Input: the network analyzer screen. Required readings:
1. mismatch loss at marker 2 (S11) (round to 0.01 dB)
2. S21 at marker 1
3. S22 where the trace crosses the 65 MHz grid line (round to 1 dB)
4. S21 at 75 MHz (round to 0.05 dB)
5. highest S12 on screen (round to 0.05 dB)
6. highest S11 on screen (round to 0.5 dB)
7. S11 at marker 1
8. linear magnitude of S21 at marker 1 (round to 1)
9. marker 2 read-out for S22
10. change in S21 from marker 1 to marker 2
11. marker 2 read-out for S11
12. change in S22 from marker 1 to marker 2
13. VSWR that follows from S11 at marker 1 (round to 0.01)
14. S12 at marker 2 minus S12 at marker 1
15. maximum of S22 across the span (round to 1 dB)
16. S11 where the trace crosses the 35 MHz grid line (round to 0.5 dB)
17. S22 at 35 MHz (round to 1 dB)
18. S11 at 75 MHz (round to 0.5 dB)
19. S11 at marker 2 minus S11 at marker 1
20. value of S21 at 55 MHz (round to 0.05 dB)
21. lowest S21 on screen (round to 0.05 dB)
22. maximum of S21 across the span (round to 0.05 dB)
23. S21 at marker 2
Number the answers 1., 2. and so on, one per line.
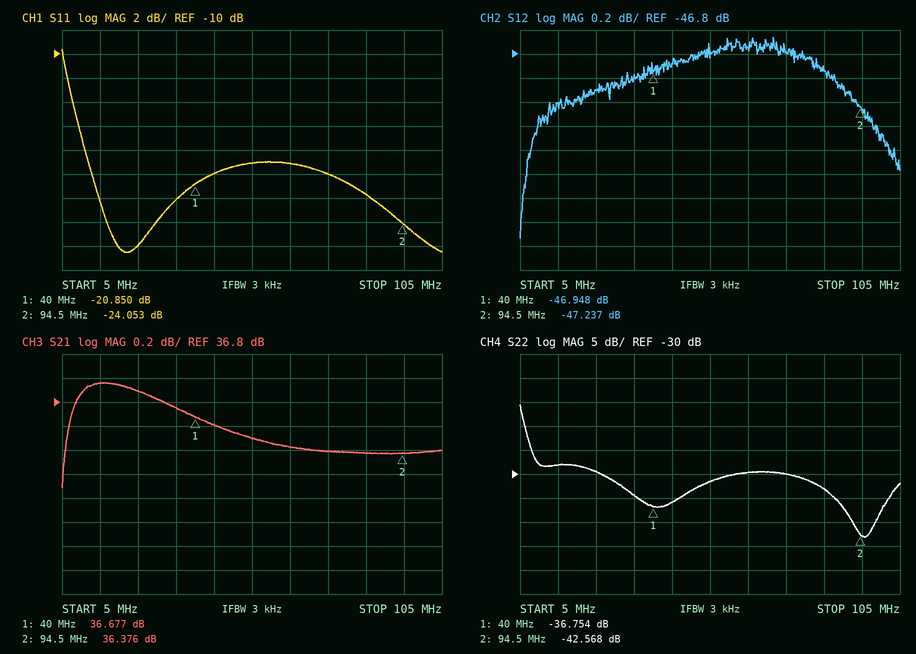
1. 0.02 dB
2. 36.677 dB
3. -30 dB
4. 36.40 dB
5. -46.65 dB
6. -9.5 dB
7. -20.850 dB
8. 68
9. -42.568 dB
10. -0.301 dB
11. -24.053 dB
12. -5.814 dB
13. 1.20
14. -0.289 dB
15. -16 dB
16. -22.0 dB
17. -34 dB
18. -20.0 dB
19. -3.203 dB
20. 36.50 dB
21. 36.10 dB
22. 36.95 dB
23. 36.376 dB
